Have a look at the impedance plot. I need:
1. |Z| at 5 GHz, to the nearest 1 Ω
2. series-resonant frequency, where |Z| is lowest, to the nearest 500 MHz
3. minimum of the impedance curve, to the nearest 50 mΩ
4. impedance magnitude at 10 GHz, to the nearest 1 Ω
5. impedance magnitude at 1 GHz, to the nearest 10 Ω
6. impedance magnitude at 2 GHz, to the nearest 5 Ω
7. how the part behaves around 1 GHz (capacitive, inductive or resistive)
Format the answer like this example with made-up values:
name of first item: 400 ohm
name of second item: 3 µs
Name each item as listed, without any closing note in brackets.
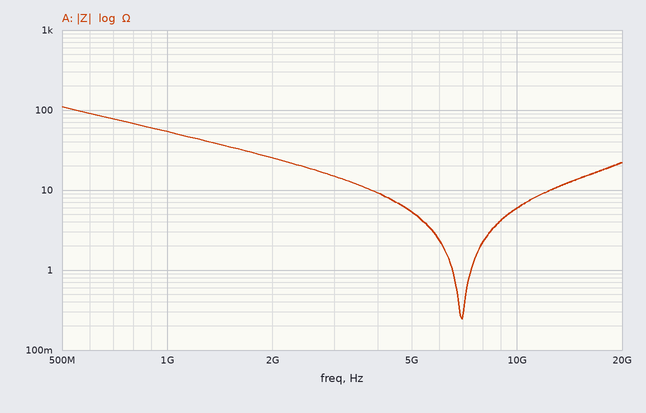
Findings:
|Z| at 5 GHz, to the nearest 1 Ω: 5 Ω
series-resonant frequency, where |Z| is lowest, to the nearest 500 MHz: 7.0 GHz
minimum of the impedance curve, to the nearest 50 mΩ: 250 mΩ
impedance magnitude at 10 GHz, to the nearest 1 Ω: 6 Ω
impedance magnitude at 1 GHz, to the nearest 10 Ω: 50 Ω
impedance magnitude at 2 GHz, to the nearest 5 Ω: 25 Ω
how the part behaves around 1 GHz: capacitive
